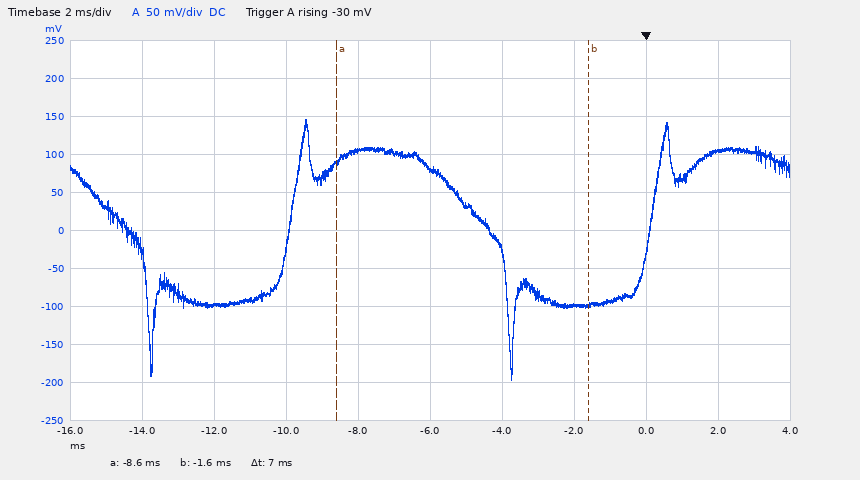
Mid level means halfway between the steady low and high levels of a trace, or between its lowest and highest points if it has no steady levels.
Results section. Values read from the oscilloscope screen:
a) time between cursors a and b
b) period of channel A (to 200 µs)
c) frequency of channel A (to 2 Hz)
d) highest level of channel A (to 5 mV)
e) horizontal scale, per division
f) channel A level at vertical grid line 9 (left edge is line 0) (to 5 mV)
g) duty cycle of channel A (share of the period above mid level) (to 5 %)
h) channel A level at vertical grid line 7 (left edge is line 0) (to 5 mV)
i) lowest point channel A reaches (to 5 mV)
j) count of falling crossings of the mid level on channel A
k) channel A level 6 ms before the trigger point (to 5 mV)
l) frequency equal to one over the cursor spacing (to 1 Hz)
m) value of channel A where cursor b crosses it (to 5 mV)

7 ms
10.0 ms
100 Hz
145 mV
2 ms
105 mV
60 %
-100 mV
-195 mV
2
80 mV
143 Hz
-100 mV
